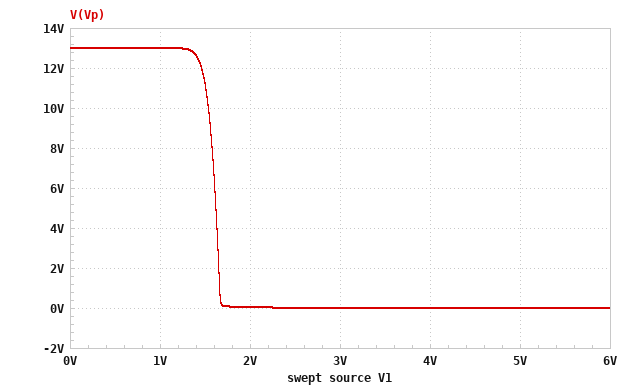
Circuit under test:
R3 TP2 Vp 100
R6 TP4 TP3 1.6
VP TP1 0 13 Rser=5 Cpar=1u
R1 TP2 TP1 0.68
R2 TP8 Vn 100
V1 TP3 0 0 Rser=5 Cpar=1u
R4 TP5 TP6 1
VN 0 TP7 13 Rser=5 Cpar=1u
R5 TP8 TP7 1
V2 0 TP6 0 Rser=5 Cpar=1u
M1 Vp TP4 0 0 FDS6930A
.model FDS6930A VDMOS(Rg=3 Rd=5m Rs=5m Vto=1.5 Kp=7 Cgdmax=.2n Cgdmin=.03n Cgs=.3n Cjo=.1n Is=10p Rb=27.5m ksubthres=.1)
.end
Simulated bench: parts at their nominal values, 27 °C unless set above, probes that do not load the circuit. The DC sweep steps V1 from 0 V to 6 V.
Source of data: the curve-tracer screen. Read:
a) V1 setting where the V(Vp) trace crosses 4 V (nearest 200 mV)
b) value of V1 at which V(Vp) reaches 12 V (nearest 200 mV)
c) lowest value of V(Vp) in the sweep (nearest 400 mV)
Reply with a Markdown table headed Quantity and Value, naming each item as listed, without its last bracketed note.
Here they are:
| Quantity | Value |
|---|---|
| V1 setting where the V(Vp) trace crosses 4 V | 1.6 V |
| value of V1 at which V(Vp) reaches 12 V | 1.4 V |
| lowest value of V(Vp) in the sweep | 0 V |
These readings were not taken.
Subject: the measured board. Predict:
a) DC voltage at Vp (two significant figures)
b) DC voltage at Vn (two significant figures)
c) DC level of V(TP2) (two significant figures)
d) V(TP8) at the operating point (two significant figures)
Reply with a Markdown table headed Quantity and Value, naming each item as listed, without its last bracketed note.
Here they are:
| Quantity | Value |
|---|---|
| DC voltage at Vp | 13 V |
| DC voltage at Vn | -13 V |
| DC level of V(TP2) | 13 V |
| V(TP8) at the operating point | -13 V |
